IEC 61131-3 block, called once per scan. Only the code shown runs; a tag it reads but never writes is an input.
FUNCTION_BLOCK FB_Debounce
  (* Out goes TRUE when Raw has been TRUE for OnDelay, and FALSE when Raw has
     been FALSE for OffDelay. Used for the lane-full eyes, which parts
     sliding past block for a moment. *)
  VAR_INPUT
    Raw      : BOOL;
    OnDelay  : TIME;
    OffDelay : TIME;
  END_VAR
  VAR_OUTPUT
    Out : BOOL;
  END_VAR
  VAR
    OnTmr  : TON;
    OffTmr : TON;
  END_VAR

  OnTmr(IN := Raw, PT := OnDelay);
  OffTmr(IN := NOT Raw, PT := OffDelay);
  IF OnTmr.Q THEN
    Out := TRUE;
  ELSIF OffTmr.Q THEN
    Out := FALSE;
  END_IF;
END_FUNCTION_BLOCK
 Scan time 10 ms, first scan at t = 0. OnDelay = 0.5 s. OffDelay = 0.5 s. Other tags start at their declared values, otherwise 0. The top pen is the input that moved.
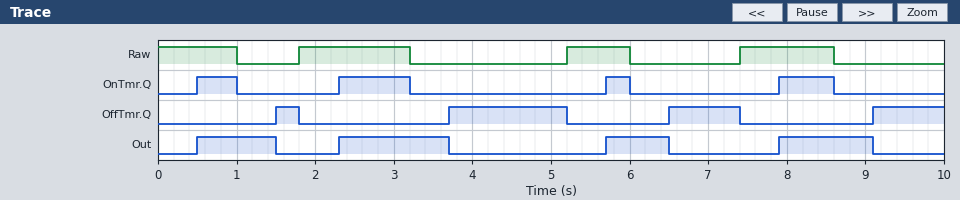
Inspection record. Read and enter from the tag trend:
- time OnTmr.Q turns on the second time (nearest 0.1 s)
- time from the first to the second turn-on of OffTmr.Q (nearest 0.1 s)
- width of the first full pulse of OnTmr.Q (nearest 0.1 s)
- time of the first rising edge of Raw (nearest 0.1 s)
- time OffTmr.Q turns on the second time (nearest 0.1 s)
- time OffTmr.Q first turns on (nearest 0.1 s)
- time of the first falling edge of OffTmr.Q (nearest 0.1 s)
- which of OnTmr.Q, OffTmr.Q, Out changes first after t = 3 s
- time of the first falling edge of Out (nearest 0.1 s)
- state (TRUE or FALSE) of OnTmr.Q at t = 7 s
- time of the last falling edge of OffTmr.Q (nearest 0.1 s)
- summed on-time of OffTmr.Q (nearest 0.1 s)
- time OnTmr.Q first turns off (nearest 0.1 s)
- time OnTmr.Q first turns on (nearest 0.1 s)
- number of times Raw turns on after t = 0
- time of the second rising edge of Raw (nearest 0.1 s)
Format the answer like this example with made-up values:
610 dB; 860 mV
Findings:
2.3 s; 2.2 s; 0.5 s; 1.8 s; 3.7 s; 1.5 s; 1.8 s; OnTmr.Q; 1.5 s; FALSE; 7.4 s; 3.6 s; 1.0 s; 0.5 s; 3; 5.2 s
